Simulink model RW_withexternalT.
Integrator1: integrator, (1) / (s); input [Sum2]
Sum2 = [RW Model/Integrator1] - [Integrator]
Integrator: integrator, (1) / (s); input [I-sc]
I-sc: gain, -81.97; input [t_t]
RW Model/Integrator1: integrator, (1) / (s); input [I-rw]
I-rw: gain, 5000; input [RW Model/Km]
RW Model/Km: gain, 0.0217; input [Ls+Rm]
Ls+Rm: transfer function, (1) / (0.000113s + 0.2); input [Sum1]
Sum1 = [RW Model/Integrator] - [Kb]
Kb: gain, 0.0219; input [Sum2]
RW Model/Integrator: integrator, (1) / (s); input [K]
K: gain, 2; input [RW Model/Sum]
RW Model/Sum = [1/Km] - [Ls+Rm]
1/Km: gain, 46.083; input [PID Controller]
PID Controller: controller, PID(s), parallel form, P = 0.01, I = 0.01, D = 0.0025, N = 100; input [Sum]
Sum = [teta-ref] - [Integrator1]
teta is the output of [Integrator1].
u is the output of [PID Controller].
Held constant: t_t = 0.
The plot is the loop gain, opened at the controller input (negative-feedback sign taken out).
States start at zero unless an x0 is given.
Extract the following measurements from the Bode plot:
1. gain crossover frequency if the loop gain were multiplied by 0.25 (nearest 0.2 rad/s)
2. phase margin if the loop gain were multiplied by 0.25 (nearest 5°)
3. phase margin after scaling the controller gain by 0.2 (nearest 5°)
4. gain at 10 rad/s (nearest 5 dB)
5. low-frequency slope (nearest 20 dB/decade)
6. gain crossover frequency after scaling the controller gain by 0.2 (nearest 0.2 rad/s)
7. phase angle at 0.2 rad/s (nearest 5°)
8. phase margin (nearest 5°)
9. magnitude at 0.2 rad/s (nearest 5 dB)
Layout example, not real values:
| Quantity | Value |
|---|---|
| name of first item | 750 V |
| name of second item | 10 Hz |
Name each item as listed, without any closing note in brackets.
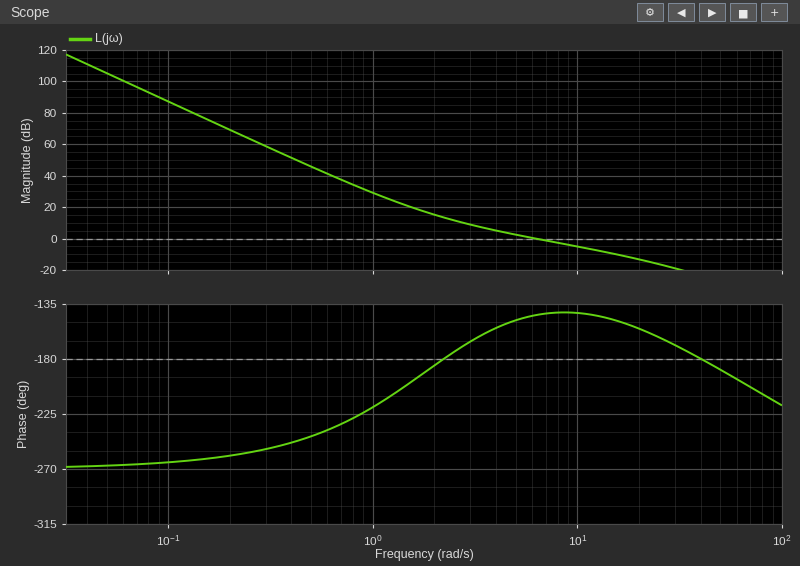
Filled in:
| Quantity | Value |
|---|---|
| gain crossover frequency if the loop gain were multiplied by 0.25 | 2.4 rad/s |
| phase margin if the loop gain were multiplied by 0.25 | 5° |
| phase margin after scaling the controller gain by 0.2 | 0° |
| gain at 10 rad/s | -5 dB |
| low-frequency slope | -60 dB/decade |
| gain crossover frequency after scaling the controller gain by 0.2 | 2.2 rad/s |
| phase angle at 0.2 rad/s | -260° |
| phase margin | 35° |
| magnitude at 0.2 rad/s | 70 dB |
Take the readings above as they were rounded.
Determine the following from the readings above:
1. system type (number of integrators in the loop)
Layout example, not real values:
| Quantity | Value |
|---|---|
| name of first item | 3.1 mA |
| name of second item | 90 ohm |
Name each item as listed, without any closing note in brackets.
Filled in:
| Quantity | Value |
|---|---|
| system type | 3 |
